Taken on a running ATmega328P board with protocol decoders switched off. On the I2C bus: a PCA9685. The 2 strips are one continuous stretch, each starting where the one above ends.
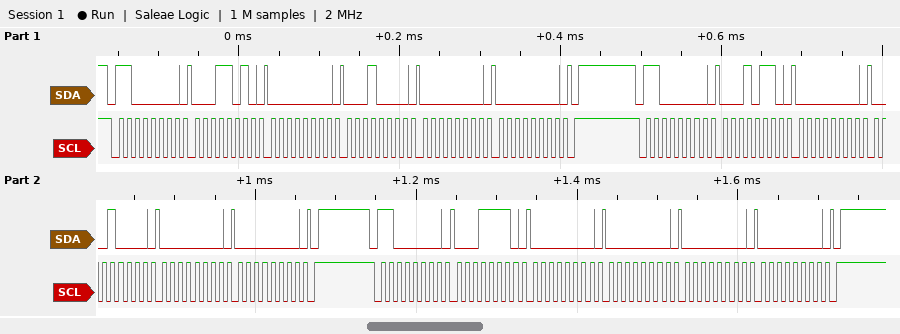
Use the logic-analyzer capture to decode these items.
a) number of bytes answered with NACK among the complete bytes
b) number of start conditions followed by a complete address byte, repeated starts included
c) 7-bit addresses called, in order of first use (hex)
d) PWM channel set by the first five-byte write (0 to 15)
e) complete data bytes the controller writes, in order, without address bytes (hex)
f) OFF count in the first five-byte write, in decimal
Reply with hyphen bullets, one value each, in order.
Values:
- 0
- 3
- 0x60
- 5
- 1A 00 10 00 00 16 00 10 00 00 1E 00 00 00 00
- 0
